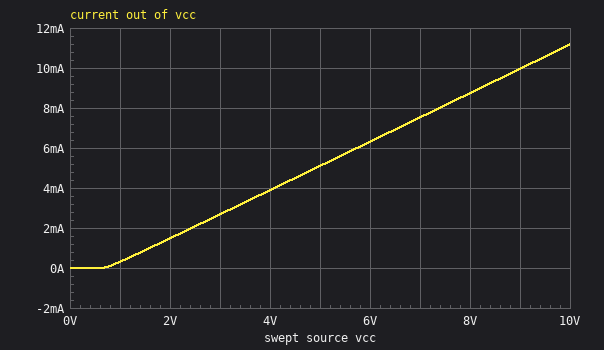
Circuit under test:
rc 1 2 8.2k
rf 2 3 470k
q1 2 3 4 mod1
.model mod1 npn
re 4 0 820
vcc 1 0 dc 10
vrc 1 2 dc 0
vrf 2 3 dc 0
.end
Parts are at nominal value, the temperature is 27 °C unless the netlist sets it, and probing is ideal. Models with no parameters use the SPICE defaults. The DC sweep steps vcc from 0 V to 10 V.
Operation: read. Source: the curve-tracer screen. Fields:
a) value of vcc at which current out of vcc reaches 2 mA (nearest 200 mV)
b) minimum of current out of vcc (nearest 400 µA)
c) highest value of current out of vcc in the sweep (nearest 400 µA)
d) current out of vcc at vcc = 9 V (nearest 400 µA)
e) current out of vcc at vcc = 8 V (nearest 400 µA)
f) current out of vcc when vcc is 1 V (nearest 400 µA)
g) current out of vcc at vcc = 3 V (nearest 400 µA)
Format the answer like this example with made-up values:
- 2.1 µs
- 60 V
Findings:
- 2.4 V
- 0 A
- 11.2 mA
- 10.0 mA
- 8.8 mA
- 400 µA
- 2.8 mA
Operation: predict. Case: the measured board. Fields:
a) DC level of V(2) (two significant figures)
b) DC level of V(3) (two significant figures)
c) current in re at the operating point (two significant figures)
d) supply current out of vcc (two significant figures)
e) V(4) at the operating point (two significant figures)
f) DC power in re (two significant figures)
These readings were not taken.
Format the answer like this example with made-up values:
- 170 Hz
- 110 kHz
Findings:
- 10 V
- 10 V
- 11 mA
- 11 mA
- 9.2 V
- 100 mW
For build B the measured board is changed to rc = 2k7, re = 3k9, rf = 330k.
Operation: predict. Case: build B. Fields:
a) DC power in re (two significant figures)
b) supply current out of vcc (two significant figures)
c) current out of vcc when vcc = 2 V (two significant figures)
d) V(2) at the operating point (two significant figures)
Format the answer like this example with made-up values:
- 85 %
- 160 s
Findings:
- 22 mW
- 2.4 mA
- 320 µA
- 10 V
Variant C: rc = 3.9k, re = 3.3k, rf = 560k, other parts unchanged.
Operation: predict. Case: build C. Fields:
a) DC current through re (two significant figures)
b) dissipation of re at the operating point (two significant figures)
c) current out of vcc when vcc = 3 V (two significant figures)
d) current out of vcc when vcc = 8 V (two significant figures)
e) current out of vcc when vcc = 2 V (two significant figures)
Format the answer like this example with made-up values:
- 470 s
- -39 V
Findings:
- 2.8 mA
- 26 mW
- 680 µA
- 2.2 mA
- 380 µA
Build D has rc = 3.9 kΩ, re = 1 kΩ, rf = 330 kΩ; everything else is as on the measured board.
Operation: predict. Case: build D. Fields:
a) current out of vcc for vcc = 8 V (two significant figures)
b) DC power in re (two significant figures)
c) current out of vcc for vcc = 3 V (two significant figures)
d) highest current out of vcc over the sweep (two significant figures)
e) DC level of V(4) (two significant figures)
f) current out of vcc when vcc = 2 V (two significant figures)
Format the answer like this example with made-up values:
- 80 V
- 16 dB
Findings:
- 7.2 mA
- 84 mW
- 2.2 mA
- 9.2 mA
- 9.2 V
- 1.2 mA
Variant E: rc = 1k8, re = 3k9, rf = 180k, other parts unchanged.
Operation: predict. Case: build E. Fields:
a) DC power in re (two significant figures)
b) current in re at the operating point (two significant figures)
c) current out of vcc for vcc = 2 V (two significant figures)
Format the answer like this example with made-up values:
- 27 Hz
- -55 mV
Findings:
- 22 mW
- 2.4 mA
- 320 µA
